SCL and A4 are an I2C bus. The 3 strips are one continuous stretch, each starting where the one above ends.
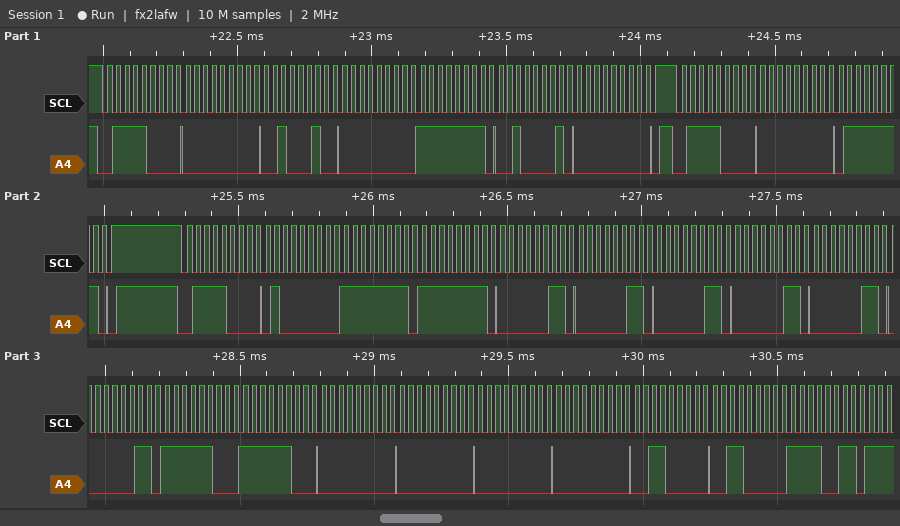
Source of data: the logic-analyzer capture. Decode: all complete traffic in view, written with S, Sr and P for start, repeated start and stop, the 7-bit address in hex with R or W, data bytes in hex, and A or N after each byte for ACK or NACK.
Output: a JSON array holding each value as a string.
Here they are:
["S 3CW A 00 A 22 A 00 A FF A 21 A 00 A P S 3CW A 00 A 7F A P S 3CW A 40 A FF A FF A 03 A 03 A 03 A 03 A 03 A 03 A FC A FC A 00 A 00 A 00 A 00 A 30 A 30 A F3 A"]
